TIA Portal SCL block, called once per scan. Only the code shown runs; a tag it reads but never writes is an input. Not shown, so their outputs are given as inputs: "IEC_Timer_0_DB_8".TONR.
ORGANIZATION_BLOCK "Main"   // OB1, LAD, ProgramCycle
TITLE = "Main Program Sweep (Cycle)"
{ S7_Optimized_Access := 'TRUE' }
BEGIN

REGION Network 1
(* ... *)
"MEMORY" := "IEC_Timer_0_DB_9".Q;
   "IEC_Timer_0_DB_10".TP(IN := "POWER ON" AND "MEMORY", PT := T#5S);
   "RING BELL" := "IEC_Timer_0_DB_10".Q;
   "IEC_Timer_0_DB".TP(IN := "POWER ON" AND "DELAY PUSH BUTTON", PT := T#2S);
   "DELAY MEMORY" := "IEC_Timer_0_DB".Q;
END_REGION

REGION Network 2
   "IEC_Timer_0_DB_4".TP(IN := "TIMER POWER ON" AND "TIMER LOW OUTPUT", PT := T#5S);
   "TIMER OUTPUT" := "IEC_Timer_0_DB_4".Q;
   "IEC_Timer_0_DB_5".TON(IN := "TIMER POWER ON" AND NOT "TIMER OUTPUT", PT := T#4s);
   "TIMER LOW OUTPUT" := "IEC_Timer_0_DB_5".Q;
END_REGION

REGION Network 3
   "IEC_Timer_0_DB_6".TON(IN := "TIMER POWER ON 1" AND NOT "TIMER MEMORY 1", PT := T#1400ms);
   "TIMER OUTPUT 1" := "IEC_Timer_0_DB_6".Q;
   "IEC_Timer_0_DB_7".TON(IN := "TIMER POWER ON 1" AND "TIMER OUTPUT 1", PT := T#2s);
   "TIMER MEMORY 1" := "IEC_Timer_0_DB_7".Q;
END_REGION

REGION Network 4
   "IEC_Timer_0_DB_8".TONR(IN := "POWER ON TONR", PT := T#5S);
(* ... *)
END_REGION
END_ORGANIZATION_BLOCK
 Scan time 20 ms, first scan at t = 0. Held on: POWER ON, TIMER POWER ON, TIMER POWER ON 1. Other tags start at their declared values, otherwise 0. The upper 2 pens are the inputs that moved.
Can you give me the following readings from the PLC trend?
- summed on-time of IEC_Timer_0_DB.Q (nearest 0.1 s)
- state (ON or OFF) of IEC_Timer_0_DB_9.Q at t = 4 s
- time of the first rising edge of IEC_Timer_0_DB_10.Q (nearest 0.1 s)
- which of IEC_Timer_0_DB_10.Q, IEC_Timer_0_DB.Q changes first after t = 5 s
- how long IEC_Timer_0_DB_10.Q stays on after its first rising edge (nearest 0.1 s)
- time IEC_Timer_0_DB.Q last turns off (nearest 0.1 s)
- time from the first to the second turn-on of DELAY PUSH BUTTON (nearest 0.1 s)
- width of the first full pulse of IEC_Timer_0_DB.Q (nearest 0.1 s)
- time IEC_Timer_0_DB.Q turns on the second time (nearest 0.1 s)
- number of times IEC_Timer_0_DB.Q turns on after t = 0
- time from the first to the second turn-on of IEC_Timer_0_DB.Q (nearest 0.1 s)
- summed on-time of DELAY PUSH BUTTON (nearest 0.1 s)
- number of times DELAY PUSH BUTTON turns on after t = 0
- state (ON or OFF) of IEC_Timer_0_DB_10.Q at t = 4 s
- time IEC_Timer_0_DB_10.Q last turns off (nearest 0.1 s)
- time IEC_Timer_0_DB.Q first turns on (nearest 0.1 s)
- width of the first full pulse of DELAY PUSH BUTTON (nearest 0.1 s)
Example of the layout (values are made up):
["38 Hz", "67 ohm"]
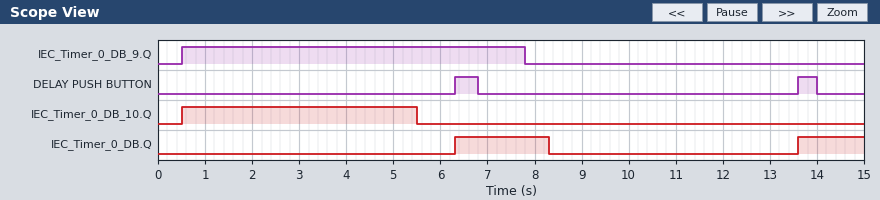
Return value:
["3.4 s", "ON", "0.5 s", "IEC_Timer_0_DB_10.Q", "5.0 s", "8.3 s", "7.3 s", "2.0 s", "13.6 s", "2", "7.3 s", "0.9 s", "2", "ON", "5.5 s", "6.3 s", "0.5 s"]
